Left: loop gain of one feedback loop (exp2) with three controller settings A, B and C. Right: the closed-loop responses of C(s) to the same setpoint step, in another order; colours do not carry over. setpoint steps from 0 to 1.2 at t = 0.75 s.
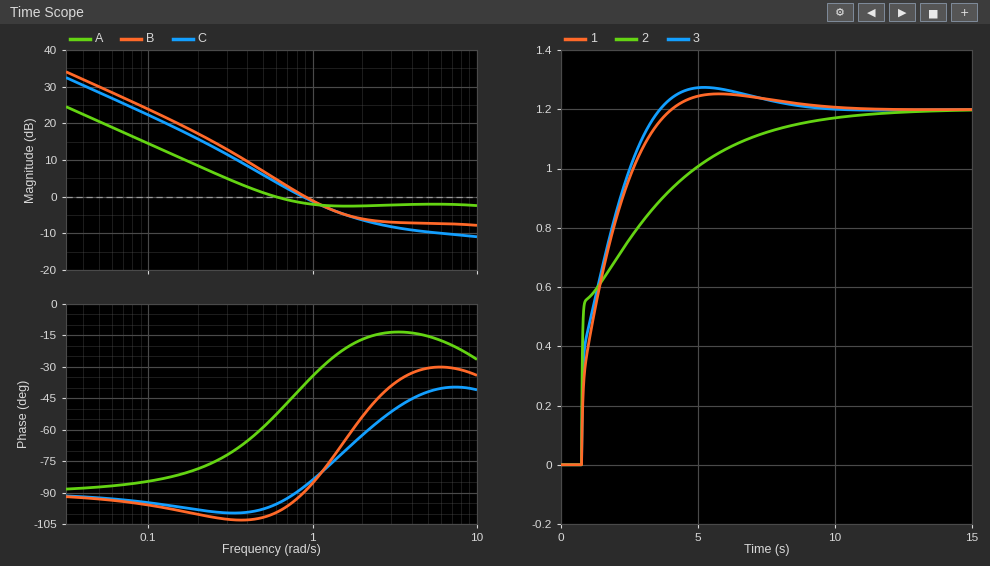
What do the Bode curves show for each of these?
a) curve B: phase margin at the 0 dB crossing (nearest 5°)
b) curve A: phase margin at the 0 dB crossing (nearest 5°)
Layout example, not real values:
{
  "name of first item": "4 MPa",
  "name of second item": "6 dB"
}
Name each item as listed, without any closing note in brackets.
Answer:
{
  "curve B: phase margin at the 0 dB crossing": "90°",
  "curve A: phase margin at the 0 dB crossing": "125°"
}
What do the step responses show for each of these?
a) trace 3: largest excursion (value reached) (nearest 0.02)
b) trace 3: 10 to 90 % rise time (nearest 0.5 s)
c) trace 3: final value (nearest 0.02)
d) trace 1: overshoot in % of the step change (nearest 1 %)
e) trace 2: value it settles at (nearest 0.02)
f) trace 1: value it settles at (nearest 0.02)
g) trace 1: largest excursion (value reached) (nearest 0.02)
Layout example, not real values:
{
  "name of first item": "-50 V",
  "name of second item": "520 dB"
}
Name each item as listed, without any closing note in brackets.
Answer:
{
  "trace 3: largest excursion (value reached)": "1.28",
  "trace 3: 10 to 90 % rise time": "2.0 s",
  "trace 3: final value": "1.20",
  "trace 1: overshoot in % of the step change": "4 %",
  "trace 2: value it settles at": "1.20",
  "trace 1: value it settles at": "1.20",
  "trace 1: largest excursion (value reached)": "1.26"
}
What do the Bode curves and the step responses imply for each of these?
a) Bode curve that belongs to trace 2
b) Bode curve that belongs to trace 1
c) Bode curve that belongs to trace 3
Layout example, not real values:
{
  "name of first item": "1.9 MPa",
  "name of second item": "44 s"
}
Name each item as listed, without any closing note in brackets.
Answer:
{
  "Bode curve that belongs to trace 2": "A",
  "Bode curve that belongs to trace 1": "C",
  "Bode curve that belongs to trace 3": "B"
}
